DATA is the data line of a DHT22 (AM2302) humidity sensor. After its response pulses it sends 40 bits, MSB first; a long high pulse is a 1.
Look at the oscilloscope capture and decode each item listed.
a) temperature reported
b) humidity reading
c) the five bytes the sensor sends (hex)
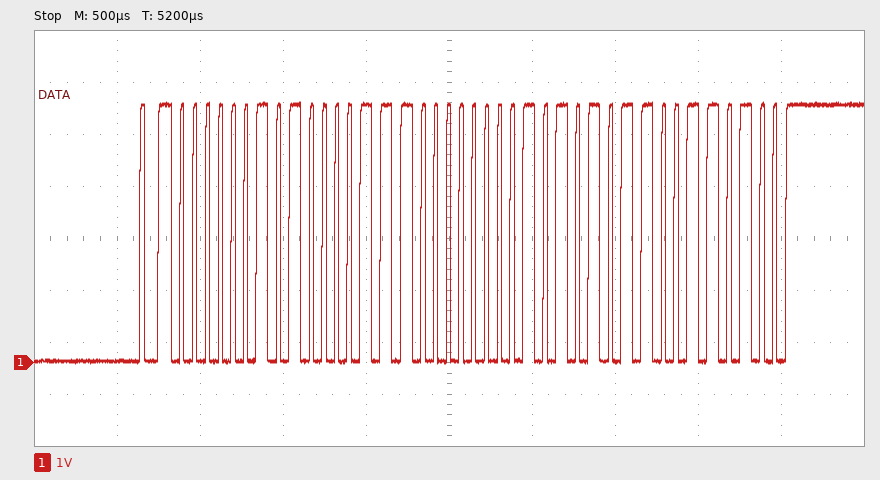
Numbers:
17.1 °C
64.7 %
02 87 00 AB 34
